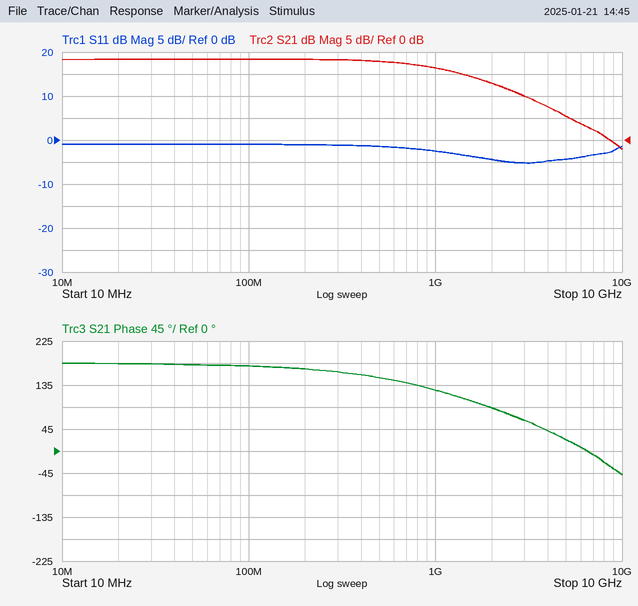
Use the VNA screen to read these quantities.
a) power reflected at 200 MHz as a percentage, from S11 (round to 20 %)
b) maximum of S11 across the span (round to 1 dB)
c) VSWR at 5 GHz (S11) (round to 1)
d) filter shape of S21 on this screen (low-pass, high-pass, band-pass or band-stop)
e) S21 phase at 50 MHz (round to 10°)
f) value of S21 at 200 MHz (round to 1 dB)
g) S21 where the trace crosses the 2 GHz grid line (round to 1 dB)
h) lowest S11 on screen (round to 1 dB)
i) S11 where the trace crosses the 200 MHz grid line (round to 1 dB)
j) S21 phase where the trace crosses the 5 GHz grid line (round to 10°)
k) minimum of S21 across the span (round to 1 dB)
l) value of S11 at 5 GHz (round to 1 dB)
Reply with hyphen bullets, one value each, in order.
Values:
- 80 %
- -1 dB
- 4
- low-pass
- 180°
- 18 dB
- 13 dB
- -5 dB
- -1 dB
- 20°
- -2 dB
- -4 dB
